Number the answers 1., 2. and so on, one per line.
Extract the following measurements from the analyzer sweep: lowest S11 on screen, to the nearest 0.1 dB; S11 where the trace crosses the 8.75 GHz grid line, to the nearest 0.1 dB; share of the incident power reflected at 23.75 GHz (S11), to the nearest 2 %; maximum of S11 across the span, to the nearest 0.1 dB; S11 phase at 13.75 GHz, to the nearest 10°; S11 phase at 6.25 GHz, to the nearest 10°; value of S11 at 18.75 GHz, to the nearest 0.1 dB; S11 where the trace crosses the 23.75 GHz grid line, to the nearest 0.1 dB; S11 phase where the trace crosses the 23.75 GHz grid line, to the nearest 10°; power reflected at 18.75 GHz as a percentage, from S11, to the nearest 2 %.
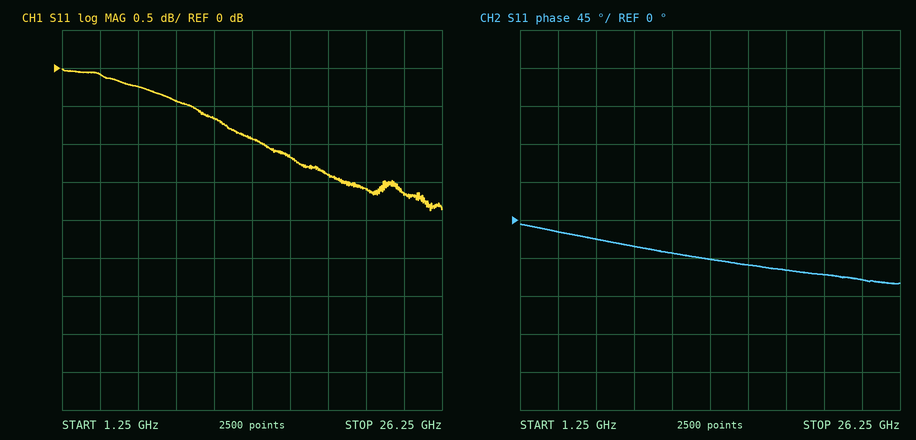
1. -1.9 dB
2. -0.4 dB
3. 68 %
4. 0.0 dB
5. -50°
6. -20°
7. -1.4 dB
8. -1.7 dB
9. -70°
10. 72 %
